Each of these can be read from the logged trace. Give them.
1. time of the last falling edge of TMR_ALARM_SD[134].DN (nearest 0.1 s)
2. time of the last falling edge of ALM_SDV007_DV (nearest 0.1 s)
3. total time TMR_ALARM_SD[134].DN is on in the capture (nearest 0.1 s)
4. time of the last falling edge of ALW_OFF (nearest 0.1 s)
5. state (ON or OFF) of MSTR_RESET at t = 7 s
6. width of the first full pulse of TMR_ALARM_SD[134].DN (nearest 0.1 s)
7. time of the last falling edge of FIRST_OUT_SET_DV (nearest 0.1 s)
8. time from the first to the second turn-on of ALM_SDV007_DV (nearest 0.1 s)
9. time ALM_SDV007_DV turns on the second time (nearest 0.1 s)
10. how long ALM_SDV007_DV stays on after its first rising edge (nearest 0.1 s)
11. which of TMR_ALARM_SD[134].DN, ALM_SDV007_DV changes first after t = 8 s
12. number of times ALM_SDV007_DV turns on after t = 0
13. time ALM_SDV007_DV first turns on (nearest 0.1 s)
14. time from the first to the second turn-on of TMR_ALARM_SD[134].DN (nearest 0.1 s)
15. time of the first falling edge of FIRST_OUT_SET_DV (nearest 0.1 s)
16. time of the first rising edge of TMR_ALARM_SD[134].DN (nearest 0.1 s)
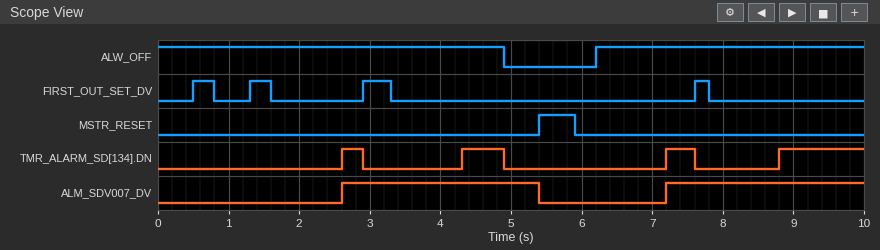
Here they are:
7.6 s
5.4 s
2.5 s
4.9 s
OFF
0.3 s
7.8 s
4.6 s
7.2 s
2.8 s
TMR_ALARM_SD[134].DN
2
2.6 s
1.7 s
0.8 s
2.6 s
